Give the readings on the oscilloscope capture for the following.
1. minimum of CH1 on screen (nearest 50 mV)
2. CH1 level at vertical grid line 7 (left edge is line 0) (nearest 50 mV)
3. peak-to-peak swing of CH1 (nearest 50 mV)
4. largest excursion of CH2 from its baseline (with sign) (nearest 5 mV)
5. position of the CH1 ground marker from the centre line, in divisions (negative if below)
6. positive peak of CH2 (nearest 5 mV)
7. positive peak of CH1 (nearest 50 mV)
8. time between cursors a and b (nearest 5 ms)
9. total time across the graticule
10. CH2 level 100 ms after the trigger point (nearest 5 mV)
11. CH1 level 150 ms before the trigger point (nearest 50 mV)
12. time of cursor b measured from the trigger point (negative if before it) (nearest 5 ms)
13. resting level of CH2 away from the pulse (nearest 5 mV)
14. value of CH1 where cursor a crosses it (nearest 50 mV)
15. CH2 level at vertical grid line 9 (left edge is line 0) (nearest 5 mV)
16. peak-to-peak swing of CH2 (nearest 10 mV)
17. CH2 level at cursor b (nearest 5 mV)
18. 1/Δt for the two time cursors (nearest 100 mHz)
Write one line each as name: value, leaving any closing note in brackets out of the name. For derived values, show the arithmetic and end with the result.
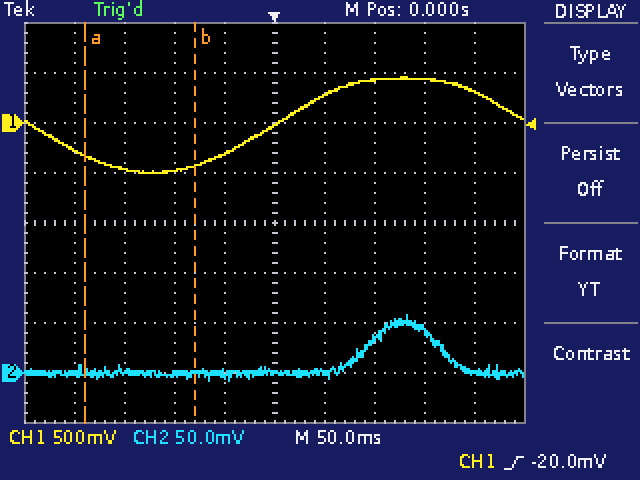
minimum of CH1 on screen: -500 mV
CH1 level at vertical grid line 7 (left edge is line 0): 450 mV
peak-to-peak swing of CH1: 450 mV − (-500 mV) = 950 mV
largest excursion of CH2 from its baseline (with sign): 60 mV − (0 mV) = +60 mV
position of the CH1 ground marker from the centre line, in divisions: +2.0 div
positive peak of CH2: 60 mV
positive peak of CH1: 450 mV
time between cursors a and b: 110 ms
total time across the graticule: 500 ms
CH2 level 100 ms after the trigger point: 35 mV
CH1 level 150 ms before the trigger point: -450 mV
time of cursor b measured from the trigger point (negative if before it): -80 ms
resting level of CH2 away from the pulse: 0 mV
value of CH1 where cursor a crosses it: -350 mV
CH2 level at vertical grid line 9 (left edge is line 0): 0 mV
peak-to-peak swing of CH2: 70 mV
CH2 level at cursor b: 0 mV
1/Δt for the two time cursors: 1 / 110 ms ≈ 9.1 Hz
